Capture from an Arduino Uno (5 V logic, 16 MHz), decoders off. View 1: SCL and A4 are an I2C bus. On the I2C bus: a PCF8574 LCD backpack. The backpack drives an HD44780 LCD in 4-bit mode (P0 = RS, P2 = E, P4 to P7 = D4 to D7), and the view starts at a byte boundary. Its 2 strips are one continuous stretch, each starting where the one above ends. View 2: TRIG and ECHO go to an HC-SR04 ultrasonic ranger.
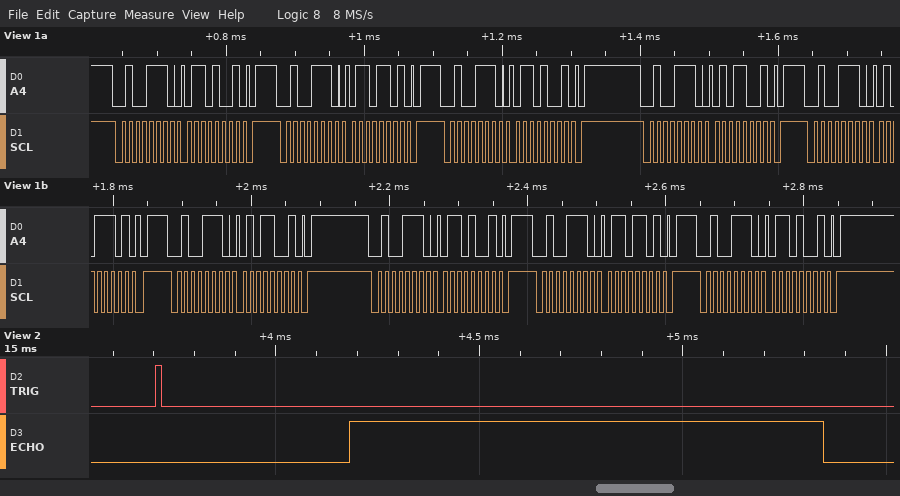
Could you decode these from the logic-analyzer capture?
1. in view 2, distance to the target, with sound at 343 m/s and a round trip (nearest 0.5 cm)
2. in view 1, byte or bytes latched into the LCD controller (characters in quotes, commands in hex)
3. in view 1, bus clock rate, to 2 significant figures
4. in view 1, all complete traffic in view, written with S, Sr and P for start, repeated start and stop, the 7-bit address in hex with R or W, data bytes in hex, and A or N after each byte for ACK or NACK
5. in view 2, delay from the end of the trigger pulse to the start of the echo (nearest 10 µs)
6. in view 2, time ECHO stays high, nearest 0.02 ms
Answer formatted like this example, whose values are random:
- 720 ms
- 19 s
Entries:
- 20 cm
- 'e'
- 100 kHz
- S 27W A 69 A P S 27W A 6D A P S 27W A 69 A P S 27W A 59 A P S 27W A 5D A P S 27W A 59 A P S 27W A 69 A P S 27W A 6D A P S 27W A 69 A P
- 460 µs
- 1.16 ms
